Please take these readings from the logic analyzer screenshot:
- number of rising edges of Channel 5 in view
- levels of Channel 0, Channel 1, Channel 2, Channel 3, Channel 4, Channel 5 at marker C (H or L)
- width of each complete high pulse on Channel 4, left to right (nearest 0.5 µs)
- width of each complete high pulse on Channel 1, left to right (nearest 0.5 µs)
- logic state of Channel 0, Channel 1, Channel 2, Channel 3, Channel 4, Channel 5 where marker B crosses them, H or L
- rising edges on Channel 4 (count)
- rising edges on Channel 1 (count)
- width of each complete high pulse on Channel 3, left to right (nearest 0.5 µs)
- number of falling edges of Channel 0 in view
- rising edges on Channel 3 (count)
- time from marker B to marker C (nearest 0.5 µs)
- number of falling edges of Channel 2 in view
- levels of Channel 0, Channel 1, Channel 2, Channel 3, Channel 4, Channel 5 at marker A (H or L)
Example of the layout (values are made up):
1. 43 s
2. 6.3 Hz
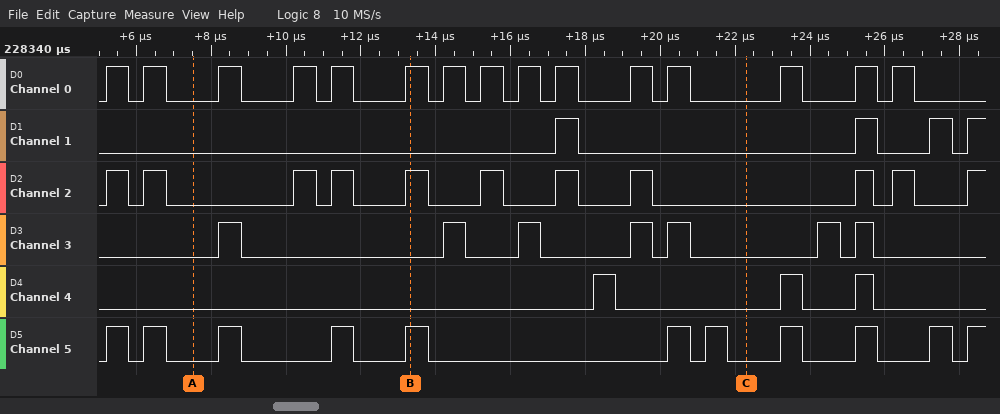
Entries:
1. 11
2. Channel 0=L, Channel 1=L, Channel 2=L, Channel 3=L, Channel 4=L, Channel 5=L
3. 0.5 µs, 0.5 µs, 0.5 µs
4. 0.5 µs, 0.5 µs, 0.5 µs
5. Channel 0=H, Channel 1=L, Channel 2=H, Channel 3=L, Channel 4=L, Channel 5=H
6. 3
7. 4
8. 0.5 µs, 0.5 µs, 0.5 µs, 0.5 µs, 0.5 µs, 0.5 µs, 0.5 µs
9. 15
10. 7
11. 9 µs
12. 10
13. Channel 0=L, Channel 1=L, Channel 2=L, Channel 3=L, Channel 4=L, Channel 5=L
